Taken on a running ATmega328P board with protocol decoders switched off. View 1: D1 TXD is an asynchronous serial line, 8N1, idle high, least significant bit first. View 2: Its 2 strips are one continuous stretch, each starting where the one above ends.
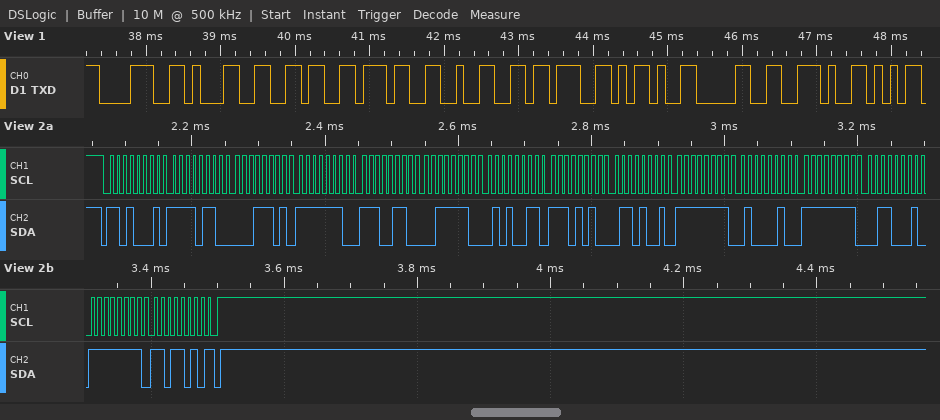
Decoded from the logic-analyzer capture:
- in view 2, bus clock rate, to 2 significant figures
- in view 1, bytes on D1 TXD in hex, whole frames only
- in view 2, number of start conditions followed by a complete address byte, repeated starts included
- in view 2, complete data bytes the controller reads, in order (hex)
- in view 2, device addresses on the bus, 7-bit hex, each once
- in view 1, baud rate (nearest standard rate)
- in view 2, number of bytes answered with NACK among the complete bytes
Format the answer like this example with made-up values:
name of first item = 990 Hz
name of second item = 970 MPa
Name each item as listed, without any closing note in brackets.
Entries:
in view 2, bus clock rate, to 2 significant figures = 100 kHz
in view 1, bytes on D1 TXD in hex, whole frames only = 38 31 36 37 32 3B 2D 30 2E
in view 2, number of start conditions followed by a complete address byte, repeated starts included = 1
in view 2, complete data bytes the controller reads, in order = F6 1D FE E6 3E 53 EA 69 FF 42 FF 31 FF DA
in view 2, device addresses on the bus, 7-bit hex, each once = 0x68
in view 1, baud rate = 9600 baud
in view 2, number of bytes answered with NACK among the complete bytes = 1
